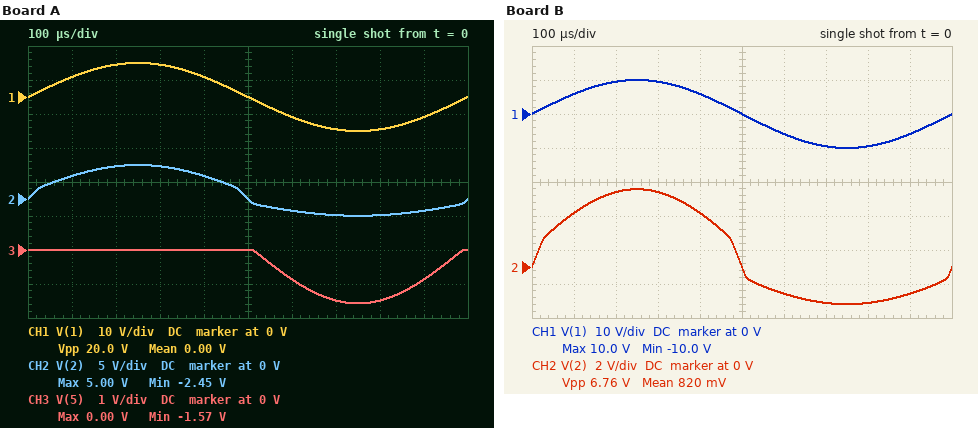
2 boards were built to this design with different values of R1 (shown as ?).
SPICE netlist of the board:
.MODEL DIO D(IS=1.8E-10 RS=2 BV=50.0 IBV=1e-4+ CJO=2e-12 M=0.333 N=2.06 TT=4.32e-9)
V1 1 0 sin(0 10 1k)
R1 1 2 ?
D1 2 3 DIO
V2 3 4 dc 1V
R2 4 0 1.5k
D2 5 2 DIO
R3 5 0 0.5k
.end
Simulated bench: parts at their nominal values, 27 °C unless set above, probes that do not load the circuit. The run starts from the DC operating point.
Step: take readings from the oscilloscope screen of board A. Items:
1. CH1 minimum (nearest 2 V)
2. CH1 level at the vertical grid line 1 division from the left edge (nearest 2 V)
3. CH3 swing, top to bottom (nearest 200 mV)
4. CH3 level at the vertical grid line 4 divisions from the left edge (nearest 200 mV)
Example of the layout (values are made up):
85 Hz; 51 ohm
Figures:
-10 V; 6 V; 1.6 V; 0 V
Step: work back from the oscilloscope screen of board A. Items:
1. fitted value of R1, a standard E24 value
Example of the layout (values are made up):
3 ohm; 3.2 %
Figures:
2.4 kΩ
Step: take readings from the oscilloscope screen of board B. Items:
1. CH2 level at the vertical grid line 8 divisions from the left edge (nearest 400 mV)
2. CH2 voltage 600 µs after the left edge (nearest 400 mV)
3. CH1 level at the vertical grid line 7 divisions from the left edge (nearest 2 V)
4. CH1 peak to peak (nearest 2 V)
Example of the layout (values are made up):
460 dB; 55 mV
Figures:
-2.0 V; -1.6 V; -10 V; 20 V
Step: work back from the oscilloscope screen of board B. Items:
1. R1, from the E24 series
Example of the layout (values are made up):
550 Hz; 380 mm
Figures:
3 kΩ
